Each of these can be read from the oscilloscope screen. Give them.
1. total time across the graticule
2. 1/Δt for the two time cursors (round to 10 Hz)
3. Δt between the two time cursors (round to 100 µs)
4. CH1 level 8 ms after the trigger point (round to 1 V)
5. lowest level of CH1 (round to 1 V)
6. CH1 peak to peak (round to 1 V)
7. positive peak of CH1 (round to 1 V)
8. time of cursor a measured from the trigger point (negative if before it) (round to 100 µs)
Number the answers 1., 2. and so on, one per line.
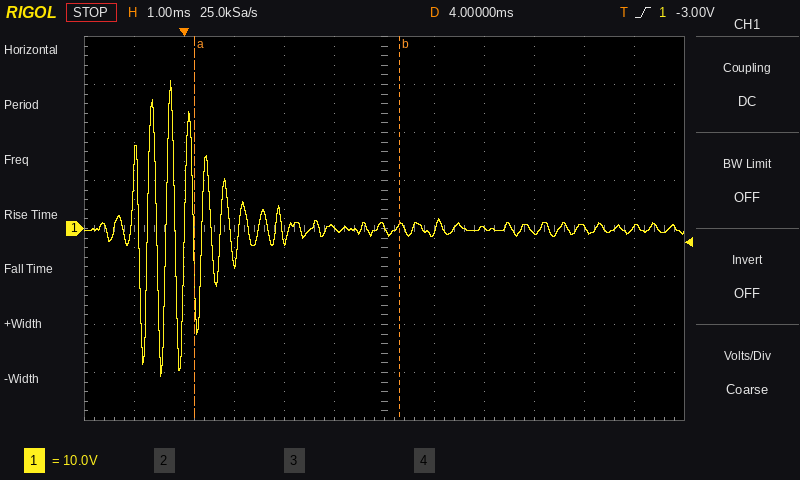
1. 12 ms
2. 240 Hz
3. 4.1 ms
4. 0 V
5. -31 V
6. 62 V
7. 31 V
8. +200 µs
